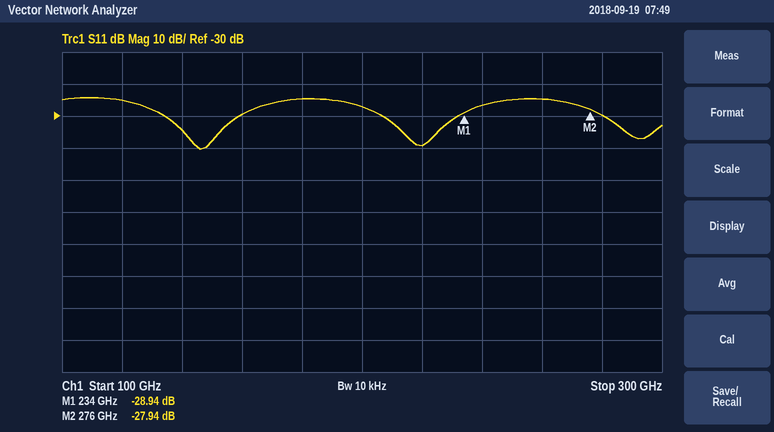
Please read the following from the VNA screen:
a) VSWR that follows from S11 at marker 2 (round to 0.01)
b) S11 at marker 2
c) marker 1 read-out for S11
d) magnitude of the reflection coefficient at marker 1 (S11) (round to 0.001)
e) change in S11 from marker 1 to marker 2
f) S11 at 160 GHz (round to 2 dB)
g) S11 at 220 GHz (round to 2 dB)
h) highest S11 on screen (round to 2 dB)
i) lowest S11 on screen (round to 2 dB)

1.08
-27.94 dB
-28.94 dB
0.036
1.00 dB
-30 dB
-40 dB
-24 dB
-40 dB
